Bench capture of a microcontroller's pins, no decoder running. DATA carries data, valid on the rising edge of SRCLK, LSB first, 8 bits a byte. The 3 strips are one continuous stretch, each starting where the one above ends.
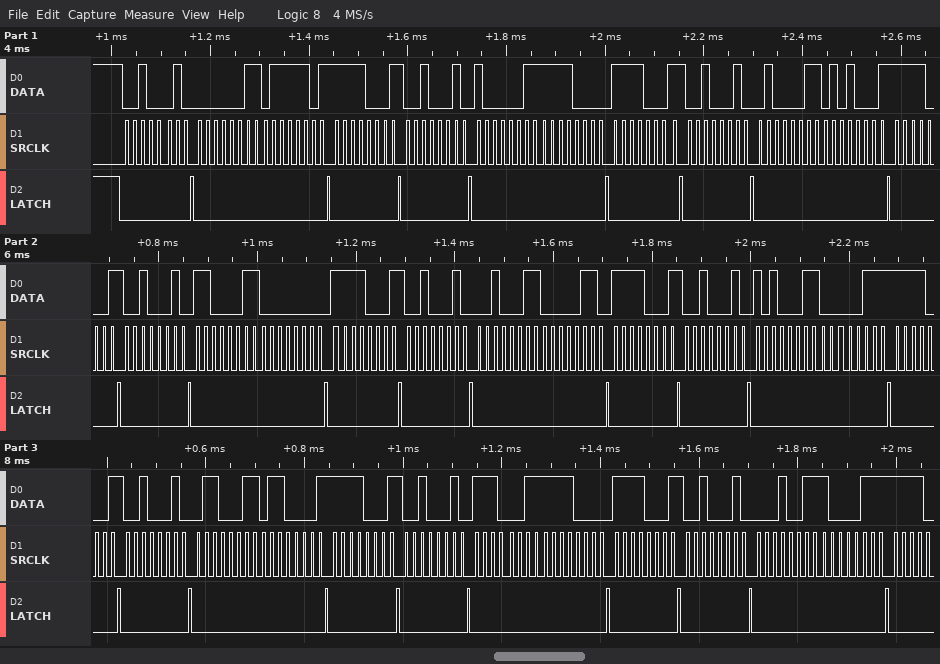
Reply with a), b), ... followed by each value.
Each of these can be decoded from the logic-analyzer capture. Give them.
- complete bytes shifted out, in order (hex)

a) 44 C0 BE 8F 44 C1 0F 8F 44 C2 8A 8F 44 C3 00 8F 44 C4 60 8F 44 C5 E0 8F 44 C6 86 8F 44 C7 0F 8F 44 C8 E1
